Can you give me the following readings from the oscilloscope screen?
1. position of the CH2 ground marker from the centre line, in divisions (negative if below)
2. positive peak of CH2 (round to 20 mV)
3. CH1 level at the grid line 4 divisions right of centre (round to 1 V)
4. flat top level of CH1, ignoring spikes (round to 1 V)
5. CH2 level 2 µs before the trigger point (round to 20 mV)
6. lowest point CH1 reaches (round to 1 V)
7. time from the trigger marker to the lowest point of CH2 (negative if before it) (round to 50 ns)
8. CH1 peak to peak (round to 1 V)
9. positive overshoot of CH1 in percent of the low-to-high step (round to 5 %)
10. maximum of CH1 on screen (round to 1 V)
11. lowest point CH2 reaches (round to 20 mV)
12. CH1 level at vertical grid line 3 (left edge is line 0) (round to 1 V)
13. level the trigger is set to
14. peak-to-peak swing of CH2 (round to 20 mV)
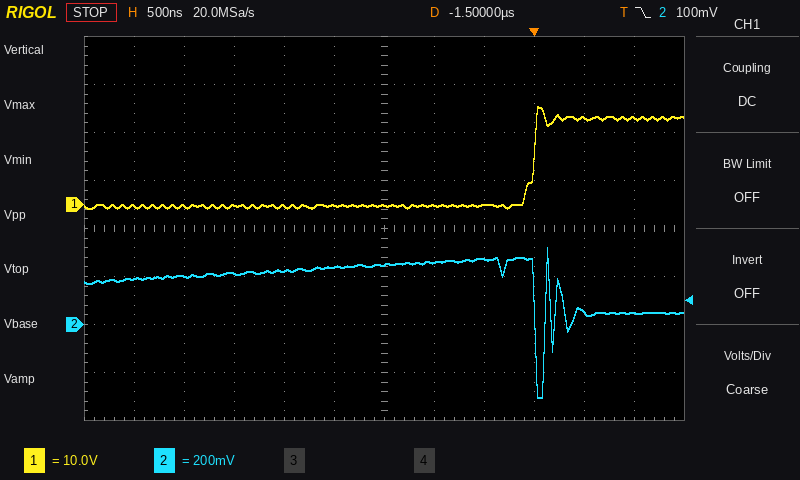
-2.0 div
320 mV
18 V
18 V
240 mV
-1 V
+50 ns
21 V
10 %
20 V
-300 mV
0 V
100 mV
620 mV
